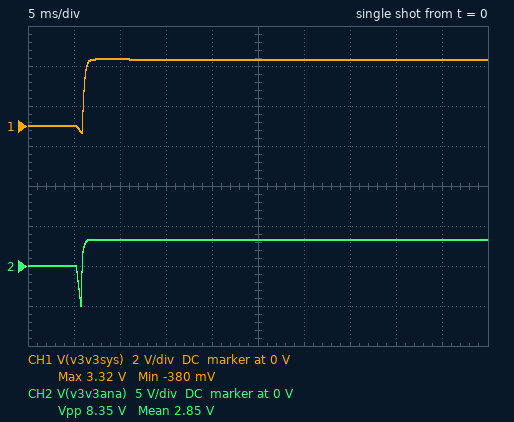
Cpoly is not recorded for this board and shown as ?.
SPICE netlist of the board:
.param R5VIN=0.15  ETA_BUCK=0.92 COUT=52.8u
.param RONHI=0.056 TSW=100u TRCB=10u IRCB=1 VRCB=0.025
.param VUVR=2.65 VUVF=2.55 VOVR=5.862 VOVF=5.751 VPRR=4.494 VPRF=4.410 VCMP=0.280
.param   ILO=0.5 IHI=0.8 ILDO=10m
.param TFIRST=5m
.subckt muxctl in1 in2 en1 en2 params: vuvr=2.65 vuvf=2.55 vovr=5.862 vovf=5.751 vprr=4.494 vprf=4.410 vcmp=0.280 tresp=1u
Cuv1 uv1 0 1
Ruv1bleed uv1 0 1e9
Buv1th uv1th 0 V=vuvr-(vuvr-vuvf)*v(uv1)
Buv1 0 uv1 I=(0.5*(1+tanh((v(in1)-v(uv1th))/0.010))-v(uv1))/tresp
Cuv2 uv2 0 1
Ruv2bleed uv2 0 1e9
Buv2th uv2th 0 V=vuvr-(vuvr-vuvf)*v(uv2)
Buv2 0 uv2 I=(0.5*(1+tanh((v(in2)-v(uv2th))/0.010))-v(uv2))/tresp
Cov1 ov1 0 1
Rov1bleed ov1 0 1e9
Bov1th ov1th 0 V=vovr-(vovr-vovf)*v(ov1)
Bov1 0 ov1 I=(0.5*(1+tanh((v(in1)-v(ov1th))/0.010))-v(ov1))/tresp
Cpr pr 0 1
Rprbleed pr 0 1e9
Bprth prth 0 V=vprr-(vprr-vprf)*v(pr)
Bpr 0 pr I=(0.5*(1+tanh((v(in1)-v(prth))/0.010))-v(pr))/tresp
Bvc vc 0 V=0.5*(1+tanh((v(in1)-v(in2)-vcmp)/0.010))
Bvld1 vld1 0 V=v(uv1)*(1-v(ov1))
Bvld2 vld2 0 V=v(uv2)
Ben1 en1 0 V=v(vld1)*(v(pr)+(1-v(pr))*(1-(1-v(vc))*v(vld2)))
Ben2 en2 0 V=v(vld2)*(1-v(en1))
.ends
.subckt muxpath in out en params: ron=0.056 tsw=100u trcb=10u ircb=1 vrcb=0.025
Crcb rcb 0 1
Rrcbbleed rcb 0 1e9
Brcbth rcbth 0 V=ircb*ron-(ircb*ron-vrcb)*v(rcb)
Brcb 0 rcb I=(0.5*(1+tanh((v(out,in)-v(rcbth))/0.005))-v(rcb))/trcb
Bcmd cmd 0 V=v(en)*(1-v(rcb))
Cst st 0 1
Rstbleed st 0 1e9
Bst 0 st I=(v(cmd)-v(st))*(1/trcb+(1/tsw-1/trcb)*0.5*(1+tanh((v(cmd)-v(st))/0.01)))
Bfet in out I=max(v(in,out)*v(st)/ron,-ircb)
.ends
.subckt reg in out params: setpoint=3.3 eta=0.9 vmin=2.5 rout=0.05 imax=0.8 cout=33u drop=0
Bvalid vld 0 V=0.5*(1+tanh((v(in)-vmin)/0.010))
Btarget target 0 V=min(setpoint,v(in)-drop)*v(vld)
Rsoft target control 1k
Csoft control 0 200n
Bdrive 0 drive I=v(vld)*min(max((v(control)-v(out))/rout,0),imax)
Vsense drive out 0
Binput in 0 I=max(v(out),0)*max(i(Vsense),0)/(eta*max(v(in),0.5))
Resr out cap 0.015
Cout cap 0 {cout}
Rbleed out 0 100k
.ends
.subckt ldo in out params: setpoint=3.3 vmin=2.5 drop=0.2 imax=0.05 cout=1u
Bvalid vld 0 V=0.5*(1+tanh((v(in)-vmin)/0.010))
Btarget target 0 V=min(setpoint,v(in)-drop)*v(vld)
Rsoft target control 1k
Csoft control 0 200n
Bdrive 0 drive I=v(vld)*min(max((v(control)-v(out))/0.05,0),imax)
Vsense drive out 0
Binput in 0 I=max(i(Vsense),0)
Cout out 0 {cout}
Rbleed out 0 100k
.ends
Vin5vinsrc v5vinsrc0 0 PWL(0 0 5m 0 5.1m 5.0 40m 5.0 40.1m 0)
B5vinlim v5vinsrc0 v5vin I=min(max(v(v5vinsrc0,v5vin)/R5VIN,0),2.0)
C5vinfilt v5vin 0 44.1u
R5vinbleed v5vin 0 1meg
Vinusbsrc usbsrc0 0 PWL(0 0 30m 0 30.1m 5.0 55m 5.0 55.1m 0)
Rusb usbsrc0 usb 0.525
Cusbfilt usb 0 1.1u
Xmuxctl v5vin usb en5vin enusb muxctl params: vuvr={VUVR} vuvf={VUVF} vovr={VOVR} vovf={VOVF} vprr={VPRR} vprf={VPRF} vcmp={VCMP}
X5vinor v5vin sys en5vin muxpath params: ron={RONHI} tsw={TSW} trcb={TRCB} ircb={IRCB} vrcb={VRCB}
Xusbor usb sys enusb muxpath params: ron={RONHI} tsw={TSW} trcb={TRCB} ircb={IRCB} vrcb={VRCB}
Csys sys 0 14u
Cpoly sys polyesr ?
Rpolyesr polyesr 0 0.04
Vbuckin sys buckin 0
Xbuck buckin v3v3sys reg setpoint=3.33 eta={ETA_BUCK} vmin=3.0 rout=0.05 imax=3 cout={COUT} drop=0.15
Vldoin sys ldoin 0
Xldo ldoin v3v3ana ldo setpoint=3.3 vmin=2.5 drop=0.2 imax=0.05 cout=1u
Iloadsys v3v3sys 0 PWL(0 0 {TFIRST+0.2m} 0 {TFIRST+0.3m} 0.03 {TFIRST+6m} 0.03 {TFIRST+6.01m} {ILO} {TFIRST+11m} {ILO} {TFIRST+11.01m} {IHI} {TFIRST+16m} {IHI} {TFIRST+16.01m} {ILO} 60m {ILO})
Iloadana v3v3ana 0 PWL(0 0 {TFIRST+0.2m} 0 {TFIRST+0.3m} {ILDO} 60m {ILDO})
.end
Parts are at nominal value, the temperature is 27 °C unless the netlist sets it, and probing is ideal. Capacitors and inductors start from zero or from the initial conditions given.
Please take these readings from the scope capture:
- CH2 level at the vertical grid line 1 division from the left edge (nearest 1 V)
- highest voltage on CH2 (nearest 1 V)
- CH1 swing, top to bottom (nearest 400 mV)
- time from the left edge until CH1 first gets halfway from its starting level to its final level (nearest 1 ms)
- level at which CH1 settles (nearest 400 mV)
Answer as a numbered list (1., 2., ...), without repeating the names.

1. 0 V
2. 3 V
3. 3.6 V
4. 6 ms
5. 3.2 V
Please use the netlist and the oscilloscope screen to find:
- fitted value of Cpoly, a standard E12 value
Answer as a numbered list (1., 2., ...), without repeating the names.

1. 560 µF
